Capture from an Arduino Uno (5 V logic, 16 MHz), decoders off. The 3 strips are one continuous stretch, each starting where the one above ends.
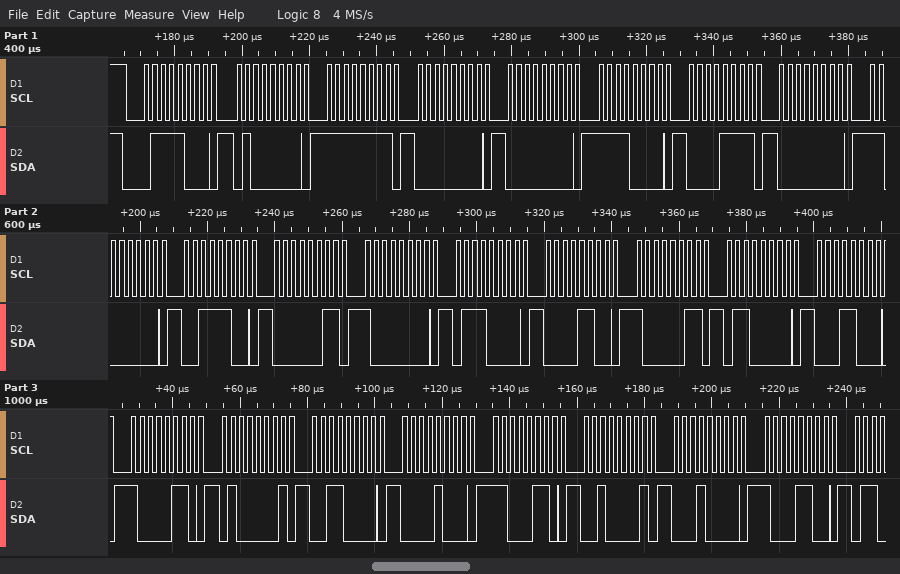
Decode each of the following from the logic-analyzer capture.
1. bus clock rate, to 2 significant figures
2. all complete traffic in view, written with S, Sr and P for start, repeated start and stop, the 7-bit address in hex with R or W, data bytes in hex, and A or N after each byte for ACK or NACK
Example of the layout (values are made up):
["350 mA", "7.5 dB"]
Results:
["400 kHz", "S 3CW A 40 A FF A 00 A 00 A F0 A 0F A 00 A C0 A 3C A 03 A 80 A 70 A 0C A 83 A 60 A 18 A 86 A 41 A 30 A 08 A C6 A 21 A 10 A 8C A"]
